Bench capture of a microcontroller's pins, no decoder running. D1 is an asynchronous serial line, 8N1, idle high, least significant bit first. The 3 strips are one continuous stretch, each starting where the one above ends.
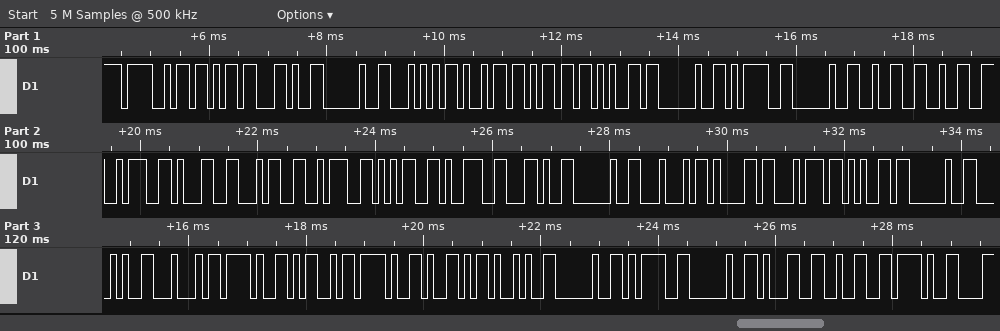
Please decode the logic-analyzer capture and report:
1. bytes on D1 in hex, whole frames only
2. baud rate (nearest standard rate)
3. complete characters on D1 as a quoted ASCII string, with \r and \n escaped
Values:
4F 6B 2C 20 54 69 6D 65 20 3D 20 32 32 3A 31 34 3A 35 39 2C 20 44 61 74 65 20 28 44 2F 4D 2F 59 29 20 3D 20 31 32 2F
9600 baud
"Ok, Time = 22:14:59, Date (D/M/Y) = 12/"
